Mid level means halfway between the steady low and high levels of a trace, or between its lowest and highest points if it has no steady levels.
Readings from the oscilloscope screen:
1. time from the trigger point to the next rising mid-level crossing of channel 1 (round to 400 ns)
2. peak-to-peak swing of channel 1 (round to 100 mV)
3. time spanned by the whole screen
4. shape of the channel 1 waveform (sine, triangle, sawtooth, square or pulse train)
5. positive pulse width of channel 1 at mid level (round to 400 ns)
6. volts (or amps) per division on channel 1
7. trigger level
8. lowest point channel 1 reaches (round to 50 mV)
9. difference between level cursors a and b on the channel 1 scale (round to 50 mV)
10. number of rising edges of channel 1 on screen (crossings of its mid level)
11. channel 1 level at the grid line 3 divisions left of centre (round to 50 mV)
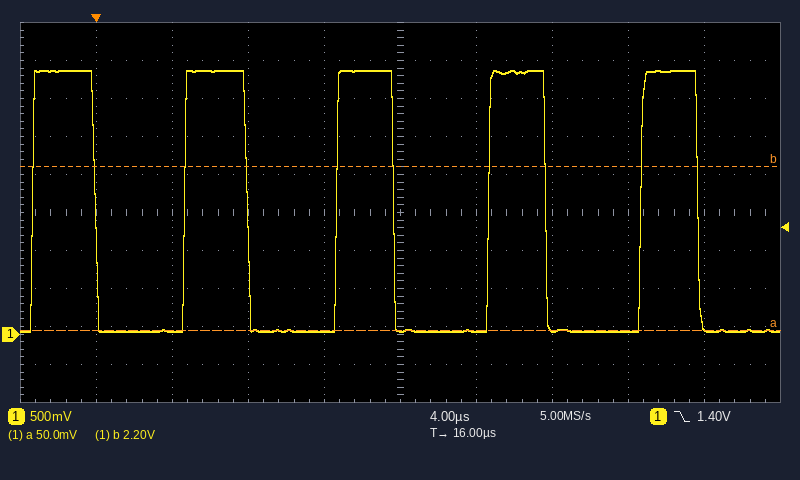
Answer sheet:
4.8 µs
3.40 V
40 µs
pulse train
3.2 µs
500 mV
1.40 V
50 mV
2.15 V
5
50 mV
